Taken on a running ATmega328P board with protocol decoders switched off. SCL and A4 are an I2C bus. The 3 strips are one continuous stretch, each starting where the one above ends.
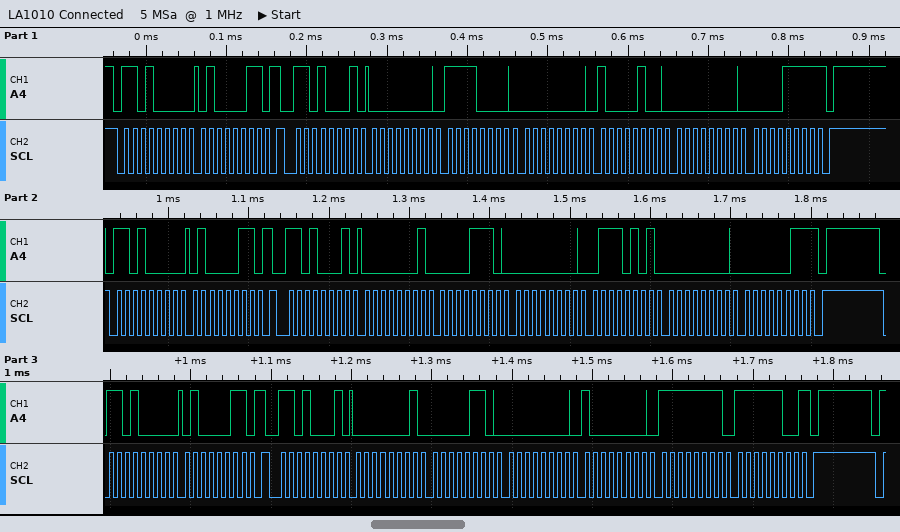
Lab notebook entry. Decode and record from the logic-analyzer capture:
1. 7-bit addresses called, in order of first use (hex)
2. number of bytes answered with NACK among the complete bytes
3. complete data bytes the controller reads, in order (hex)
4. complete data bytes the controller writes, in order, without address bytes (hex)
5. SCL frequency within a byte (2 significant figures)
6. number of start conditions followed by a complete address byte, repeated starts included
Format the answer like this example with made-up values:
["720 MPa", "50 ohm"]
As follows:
["0x68", "3", "00 F0 00 84 00 0F 01 0E 00 75 00 03 01 06 00 80 FF FC", "43 43 43", "100 kHz", "6"]
